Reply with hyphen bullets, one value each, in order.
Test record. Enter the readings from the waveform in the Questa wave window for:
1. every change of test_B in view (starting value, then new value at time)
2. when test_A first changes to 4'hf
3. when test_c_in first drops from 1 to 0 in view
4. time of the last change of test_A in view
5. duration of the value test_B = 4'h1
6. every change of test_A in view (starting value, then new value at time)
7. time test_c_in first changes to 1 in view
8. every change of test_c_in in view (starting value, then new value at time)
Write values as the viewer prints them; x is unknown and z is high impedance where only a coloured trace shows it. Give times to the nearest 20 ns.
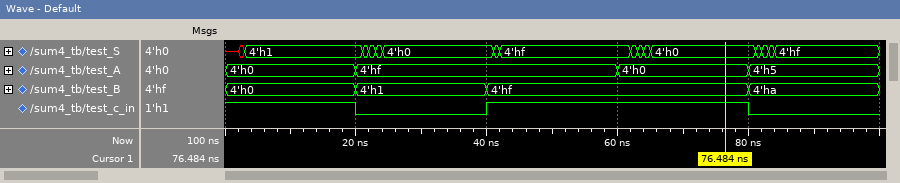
- 4'h0, 4'h1 at 20 ns, 4'hf at 40 ns, 4'ha at 80 ns
- 20 ns
- 20 ns
- 80 ns
- 20 ns
- 4'h0, 4'hf at 20 ns, 4'h0 at 60 ns, 4'h5 at 80 ns
- 40 ns
- 1, 0 at 20 ns, 1 at 40 ns, 0 at 80 ns
